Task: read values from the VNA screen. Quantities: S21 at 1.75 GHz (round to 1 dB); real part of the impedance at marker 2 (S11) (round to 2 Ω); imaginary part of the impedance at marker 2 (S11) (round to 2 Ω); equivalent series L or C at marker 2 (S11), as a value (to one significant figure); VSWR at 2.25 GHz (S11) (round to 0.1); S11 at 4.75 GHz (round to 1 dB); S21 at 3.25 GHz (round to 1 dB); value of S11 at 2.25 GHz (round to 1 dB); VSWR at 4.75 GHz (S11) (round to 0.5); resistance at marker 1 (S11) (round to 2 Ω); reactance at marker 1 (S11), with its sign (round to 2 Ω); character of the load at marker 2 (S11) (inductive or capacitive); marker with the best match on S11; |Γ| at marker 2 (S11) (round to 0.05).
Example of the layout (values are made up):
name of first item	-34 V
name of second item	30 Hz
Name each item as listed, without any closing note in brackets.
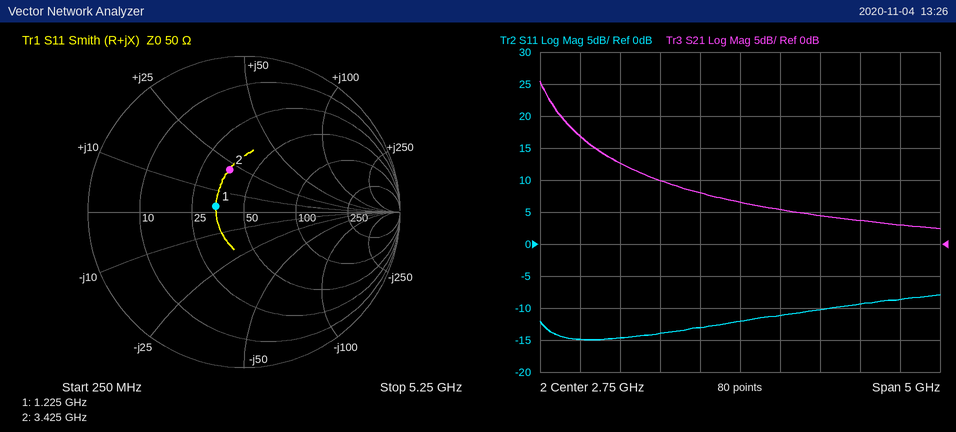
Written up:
S21 at 1.75 GHz	10 dB
real part of the impedance at marker 2 (S11)	36 Ω
imaginary part of the impedance at marker 2 (S11)	+22 Ω
equivalent series L or C at marker 2 (S11), as a value	1.0 nH
VSWR at 2.25 GHz (S11)	1.6
S11 at 4.75 GHz	-9 dB
S21 at 3.25 GHz	5 dB
value of S11 at 2.25 GHz	-13 dB
VSWR at 4.75 GHz (S11)	2.0
resistance at marker 1 (S11)	34 Ω
reactance at marker 1 (S11), with its sign	+2 Ω
character of the load at marker 2 (S11)	inductive
marker with the best match on S11	marker 1
|Γ| at marker 2 (S11)	0.30
